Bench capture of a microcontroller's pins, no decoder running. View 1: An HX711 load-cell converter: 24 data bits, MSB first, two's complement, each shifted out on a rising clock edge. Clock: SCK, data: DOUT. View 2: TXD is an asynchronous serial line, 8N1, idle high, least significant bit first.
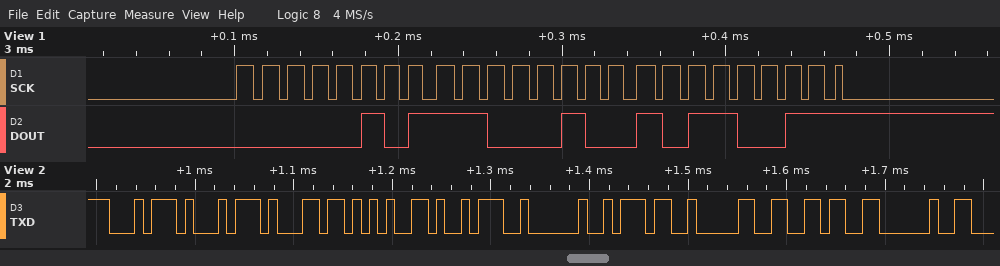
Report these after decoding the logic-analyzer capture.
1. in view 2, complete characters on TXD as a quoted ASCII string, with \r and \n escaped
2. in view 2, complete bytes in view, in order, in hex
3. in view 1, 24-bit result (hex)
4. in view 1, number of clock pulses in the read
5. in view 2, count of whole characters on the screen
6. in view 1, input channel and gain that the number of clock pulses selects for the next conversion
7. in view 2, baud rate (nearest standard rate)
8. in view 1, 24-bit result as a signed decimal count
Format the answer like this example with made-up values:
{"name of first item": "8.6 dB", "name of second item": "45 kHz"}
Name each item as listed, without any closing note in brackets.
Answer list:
{"in view 2, complete characters on TXD as a quoted ASCII string, with \\r and \\n escaped": "\"ttle: 706 \"", "in view 2, complete bytes in view, in order, in hex": "74 74 6C 65 3A 20 37 30 36 20", "in view 1, 24-bit result": "0x05C4B3", "in view 1, number of clock pulses in the read": "25", "in view 2, count of whole characters on the screen": "10", "in view 1, input channel and gain that the number of clock pulses selects for the next conversion": "channel A, gain 128", "in view 2, baud rate": "115200 baud", "in view 1, 24-bit result as a signed decimal count": "378035"}
